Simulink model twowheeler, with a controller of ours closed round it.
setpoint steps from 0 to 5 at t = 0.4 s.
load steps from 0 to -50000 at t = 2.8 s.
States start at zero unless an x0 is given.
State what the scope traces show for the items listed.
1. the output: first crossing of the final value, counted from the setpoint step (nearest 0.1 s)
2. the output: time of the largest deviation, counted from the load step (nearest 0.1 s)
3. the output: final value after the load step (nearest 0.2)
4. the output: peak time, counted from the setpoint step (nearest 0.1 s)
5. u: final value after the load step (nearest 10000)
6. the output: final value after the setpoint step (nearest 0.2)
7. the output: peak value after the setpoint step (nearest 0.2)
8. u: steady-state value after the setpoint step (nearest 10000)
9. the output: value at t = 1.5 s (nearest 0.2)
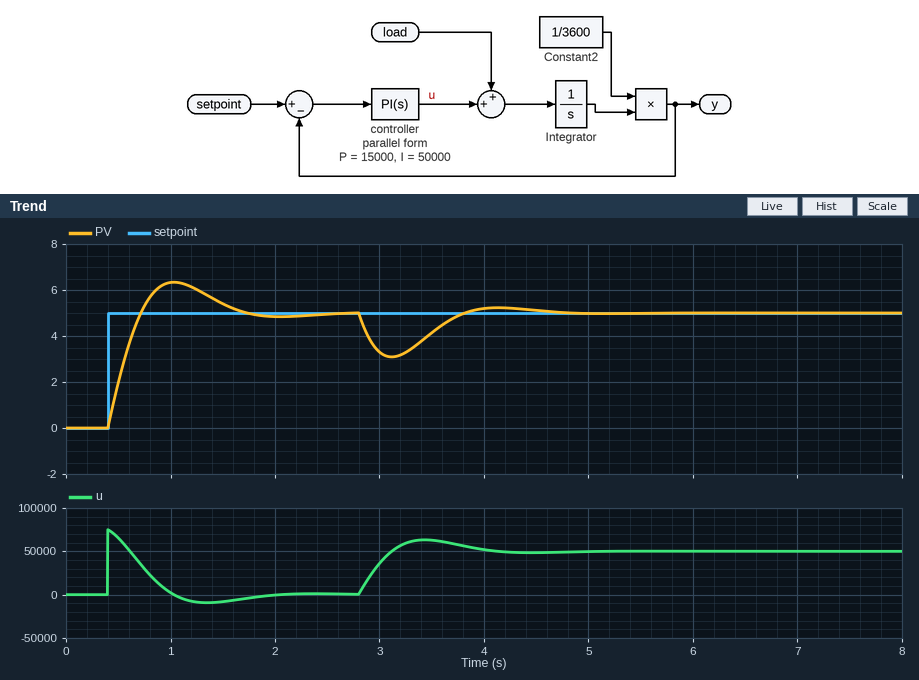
0.3 s
0.3 s
5.0
0.6 s
50000
5.0
6.4
0
5.4
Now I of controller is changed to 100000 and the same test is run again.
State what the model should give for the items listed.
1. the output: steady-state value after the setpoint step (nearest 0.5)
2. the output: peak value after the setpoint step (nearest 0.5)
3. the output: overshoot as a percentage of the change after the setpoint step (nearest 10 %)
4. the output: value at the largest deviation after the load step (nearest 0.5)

5.0
7.0
40 %
3.5
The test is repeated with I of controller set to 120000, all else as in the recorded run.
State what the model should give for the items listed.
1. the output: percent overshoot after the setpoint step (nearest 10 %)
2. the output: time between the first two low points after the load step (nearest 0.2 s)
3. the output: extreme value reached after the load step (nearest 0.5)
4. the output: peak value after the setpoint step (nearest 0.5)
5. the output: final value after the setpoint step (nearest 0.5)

40 %
1.2 s
3.5
7.0
5.0
